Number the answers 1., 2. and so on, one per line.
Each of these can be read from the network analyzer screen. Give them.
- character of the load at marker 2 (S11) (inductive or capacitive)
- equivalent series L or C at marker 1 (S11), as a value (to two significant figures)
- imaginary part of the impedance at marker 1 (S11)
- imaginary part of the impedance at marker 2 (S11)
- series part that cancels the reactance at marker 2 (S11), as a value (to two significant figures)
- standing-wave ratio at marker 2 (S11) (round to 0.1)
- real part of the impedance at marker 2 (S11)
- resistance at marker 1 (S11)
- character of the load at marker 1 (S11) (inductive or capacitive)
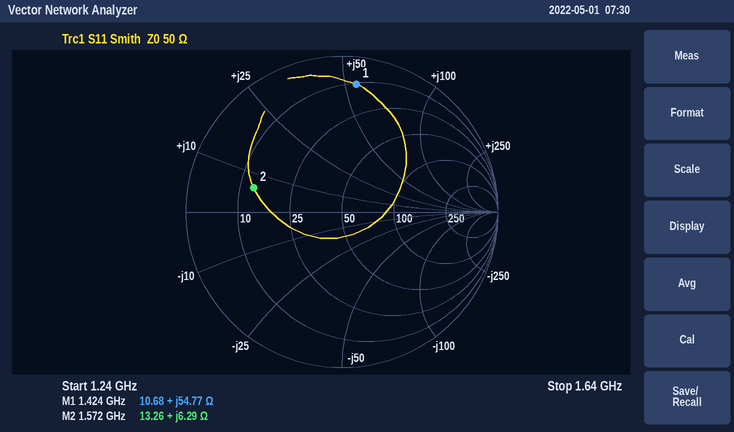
1. inductive
2. 6.1 nH
3. +54.77 Ω
4. +6.29 Ω
5. 16 pF
6. 3.8
7. 13.26 Ω
8. 10.68 Ω
9. inductive
